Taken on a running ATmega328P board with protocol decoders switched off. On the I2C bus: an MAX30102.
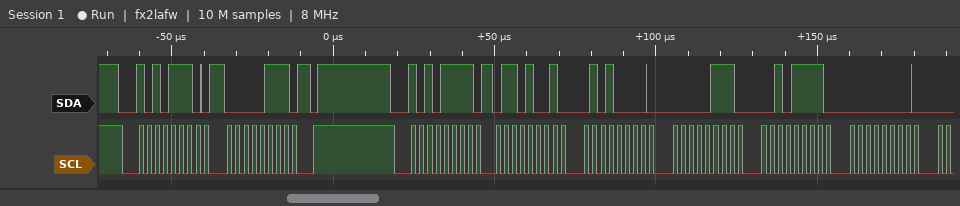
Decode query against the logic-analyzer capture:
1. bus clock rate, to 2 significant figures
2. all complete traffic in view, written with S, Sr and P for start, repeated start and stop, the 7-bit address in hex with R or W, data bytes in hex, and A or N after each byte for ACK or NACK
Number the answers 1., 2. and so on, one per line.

1. 400 kHz
2. S 57W A 07 A P S 57R A 69 A 50 A 07 A 2F A 00 A
